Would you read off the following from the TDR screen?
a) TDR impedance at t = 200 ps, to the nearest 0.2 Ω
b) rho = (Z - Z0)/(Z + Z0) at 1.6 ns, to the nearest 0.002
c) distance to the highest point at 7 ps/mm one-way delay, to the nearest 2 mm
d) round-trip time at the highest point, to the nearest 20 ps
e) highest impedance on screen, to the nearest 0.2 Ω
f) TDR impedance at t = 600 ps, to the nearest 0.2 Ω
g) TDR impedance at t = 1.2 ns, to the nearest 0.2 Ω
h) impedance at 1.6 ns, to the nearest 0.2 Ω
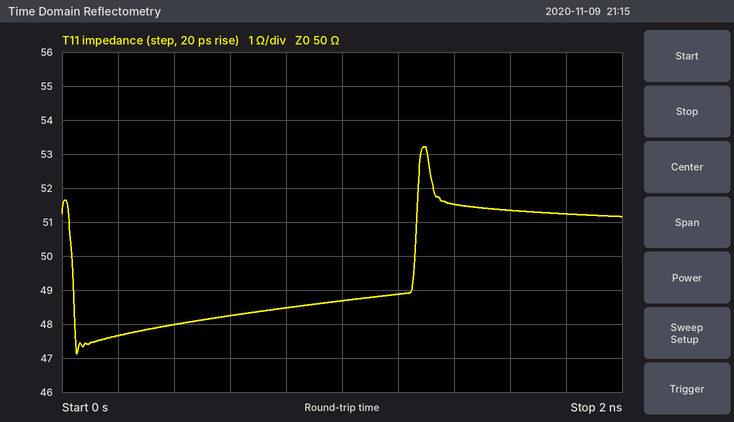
47.6 Ω
+0.014
92 mm
1.30 ns
53.2 Ω
48.2 Ω
48.8 Ω
51.4 Ω
